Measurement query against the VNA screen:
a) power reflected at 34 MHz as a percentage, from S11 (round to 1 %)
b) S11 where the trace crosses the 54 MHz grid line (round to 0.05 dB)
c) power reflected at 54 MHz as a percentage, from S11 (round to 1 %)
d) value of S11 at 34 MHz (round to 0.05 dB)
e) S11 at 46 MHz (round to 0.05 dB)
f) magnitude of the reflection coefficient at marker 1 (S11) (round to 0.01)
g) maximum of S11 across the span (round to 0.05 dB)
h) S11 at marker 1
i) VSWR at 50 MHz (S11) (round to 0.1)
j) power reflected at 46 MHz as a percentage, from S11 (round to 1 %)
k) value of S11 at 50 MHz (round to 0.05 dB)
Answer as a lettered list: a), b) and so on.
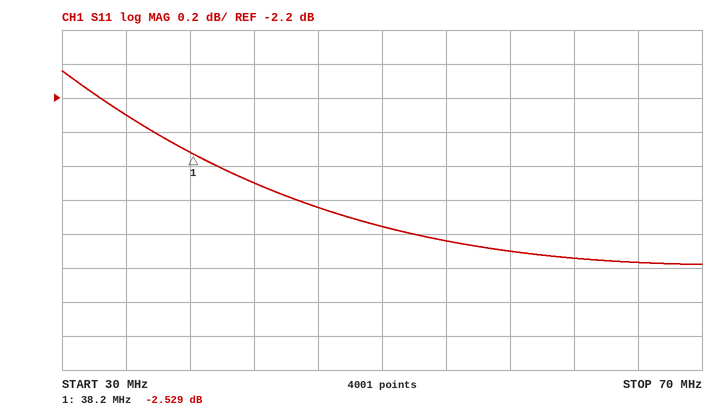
a) 59 %
b) -3.05 dB
c) 50 %
d) -2.30 dB
e) -2.85 dB
f) 0.75
g) -2.05 dB
h) -2.529 dB
i) 5.9
j) 52 %
k) -2.95 dB
